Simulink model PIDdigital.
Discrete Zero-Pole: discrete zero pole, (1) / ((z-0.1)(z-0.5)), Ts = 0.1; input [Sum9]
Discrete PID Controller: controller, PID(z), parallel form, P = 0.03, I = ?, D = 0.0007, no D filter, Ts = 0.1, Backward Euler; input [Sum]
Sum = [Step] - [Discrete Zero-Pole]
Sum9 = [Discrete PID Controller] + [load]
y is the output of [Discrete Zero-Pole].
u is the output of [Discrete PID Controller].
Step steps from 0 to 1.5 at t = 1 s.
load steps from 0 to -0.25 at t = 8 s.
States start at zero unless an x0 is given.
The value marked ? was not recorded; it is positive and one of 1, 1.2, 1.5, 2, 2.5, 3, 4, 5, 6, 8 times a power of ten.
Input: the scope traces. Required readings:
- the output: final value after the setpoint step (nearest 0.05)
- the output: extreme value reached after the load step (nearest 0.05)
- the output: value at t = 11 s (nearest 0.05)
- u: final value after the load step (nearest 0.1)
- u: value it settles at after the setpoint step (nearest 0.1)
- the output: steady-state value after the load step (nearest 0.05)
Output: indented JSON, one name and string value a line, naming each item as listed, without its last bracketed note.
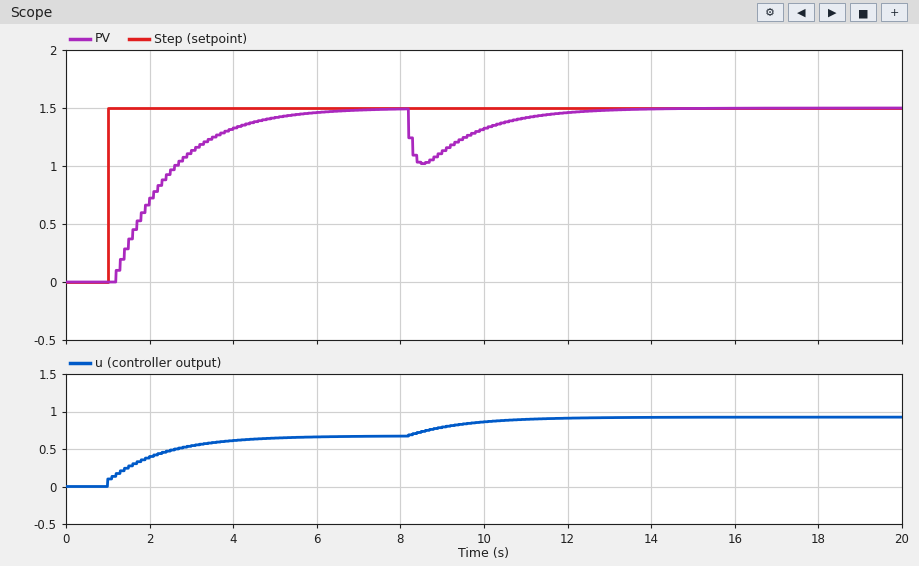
{
  "the output: final value after the setpoint step": "1.50",
  "the output: extreme value reached after the load step": "1.00",
  "the output: value at t = 11 s": "1.40",
  "u: final value after the load step": "0.9",
  "u: value it settles at after the setpoint step": "0.7",
  "the output: steady-state value after the load step": "1.50"
}
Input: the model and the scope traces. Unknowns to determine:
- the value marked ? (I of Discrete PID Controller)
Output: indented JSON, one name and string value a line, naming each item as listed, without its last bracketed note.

{
  "the value marked ?": "0.3"
}
